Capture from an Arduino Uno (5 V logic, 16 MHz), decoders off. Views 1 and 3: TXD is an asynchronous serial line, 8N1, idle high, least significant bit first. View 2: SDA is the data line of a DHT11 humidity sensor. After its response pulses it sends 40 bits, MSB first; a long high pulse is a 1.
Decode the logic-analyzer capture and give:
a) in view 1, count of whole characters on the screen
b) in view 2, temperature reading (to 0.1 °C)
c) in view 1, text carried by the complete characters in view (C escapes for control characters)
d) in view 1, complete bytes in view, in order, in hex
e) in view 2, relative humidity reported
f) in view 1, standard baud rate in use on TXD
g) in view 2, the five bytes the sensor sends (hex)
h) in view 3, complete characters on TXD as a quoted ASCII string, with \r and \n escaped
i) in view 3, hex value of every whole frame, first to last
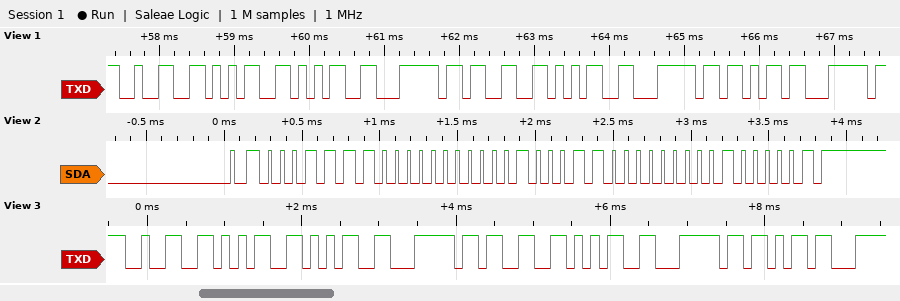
9
35.0 °C
"255|35|k|"
32 35 35 7C 33 35 7C 6B 7C
30 %
9600 baud
1E 00 23 00 41
"255|35|k"
32 35 35 7C 33 35 7C 6B
